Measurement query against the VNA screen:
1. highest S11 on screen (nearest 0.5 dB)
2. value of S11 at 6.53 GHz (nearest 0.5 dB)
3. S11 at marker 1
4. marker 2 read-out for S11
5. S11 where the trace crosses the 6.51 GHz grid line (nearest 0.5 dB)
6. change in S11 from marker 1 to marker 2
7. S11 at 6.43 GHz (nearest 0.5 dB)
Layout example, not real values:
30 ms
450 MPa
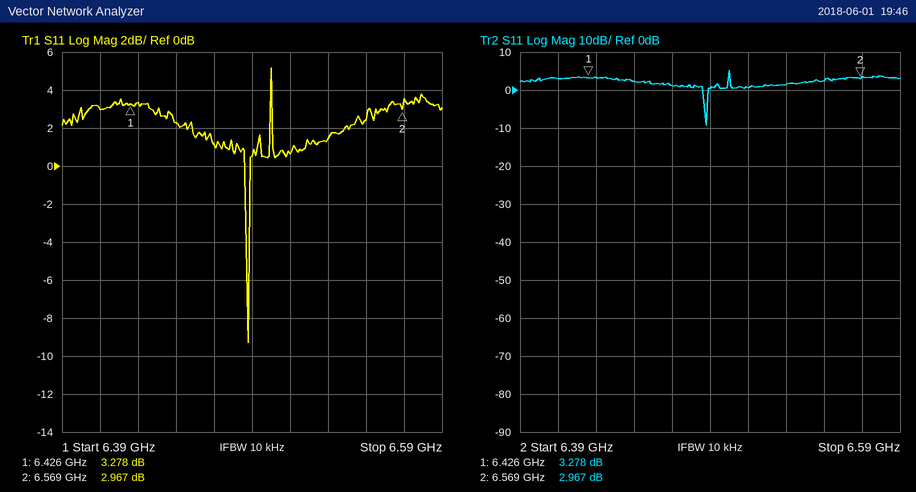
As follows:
5.0 dB
1.5 dB
3.278 dB
2.967 dB
0.5 dB
-0.311 dB
3.5 dB
